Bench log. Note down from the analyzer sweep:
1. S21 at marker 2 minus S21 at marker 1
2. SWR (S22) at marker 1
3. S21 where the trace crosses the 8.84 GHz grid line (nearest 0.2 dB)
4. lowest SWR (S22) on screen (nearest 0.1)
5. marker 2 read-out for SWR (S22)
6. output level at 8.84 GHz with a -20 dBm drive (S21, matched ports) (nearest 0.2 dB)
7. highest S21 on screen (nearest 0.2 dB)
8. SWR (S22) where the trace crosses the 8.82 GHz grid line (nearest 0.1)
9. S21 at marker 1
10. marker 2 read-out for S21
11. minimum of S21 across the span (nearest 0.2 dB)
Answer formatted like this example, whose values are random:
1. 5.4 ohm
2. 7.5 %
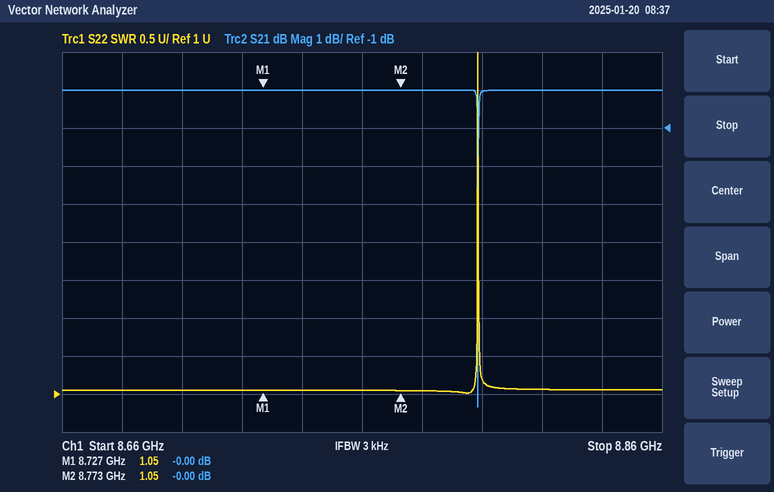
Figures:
1. 0.00 dB
2. 1.05
3. 0.0 dB
4. 1.0
5. 1.05
6. -20.0 dBm
7. 0.0 dB
8. 1.1
9. -0.00 dB
10. -0.00 dB
11. -8.4 dB
